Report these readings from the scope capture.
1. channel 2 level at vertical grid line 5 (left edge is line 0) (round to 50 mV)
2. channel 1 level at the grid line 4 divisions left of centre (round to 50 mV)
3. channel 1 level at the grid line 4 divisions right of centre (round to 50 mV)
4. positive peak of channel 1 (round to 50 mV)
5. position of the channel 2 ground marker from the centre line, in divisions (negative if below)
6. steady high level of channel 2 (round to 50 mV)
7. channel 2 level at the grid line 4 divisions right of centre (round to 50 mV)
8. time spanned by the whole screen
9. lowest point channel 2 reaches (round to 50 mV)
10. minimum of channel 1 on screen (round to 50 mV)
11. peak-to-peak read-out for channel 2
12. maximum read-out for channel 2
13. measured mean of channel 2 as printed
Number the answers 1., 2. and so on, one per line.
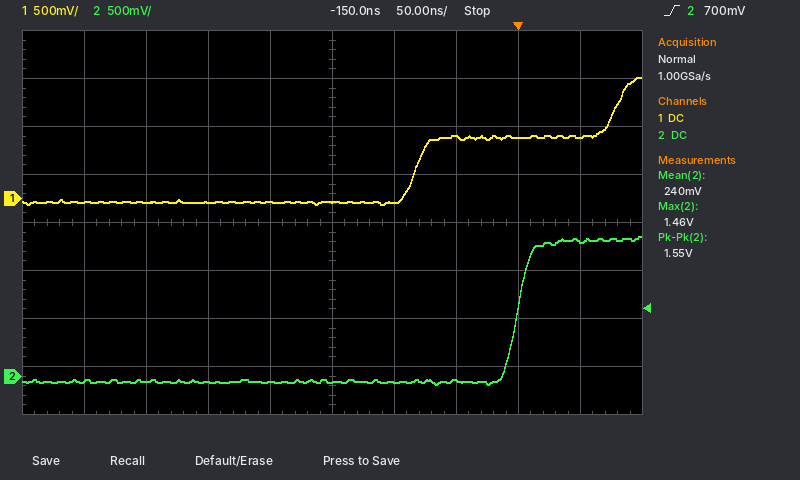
1. -50 mV
2. -50 mV
3. 650 mV
4. 1.25 V
5. -3.2 div
6. 1.40 V
7. 1.40 V
8. 500 ns
9. -100 mV
10. -50 mV
11. 1.55 V
12. 1.46 V
13. 240 mV
